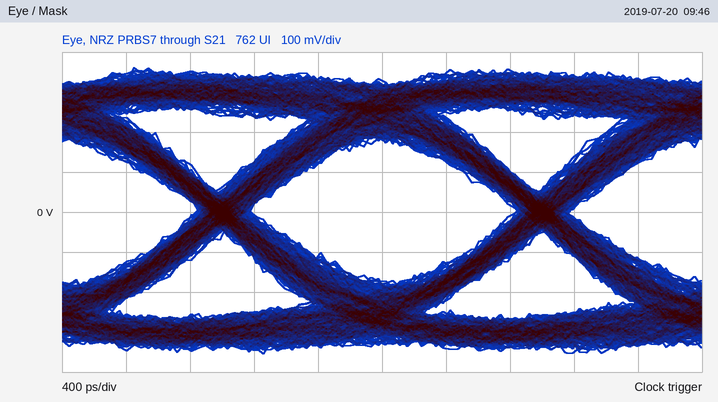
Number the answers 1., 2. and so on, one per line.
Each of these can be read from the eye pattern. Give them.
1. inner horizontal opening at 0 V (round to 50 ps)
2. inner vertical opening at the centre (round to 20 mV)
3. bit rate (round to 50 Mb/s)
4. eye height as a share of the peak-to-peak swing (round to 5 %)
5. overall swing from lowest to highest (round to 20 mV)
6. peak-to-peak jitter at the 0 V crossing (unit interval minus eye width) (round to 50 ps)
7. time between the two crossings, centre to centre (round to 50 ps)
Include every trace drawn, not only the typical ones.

1. 1.65 ns
2. 360 mV
3. 500 Mb/s
4. 50 %
5. 720 mV
6. 350 ps
7. 2.00 ns
